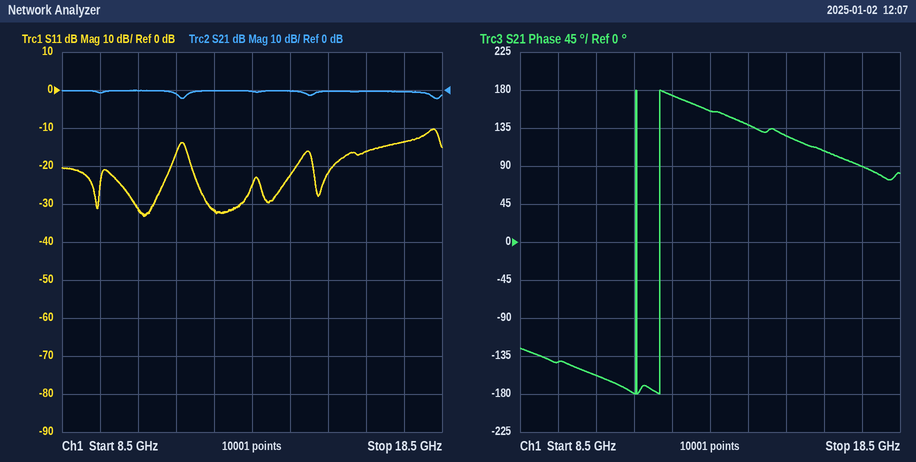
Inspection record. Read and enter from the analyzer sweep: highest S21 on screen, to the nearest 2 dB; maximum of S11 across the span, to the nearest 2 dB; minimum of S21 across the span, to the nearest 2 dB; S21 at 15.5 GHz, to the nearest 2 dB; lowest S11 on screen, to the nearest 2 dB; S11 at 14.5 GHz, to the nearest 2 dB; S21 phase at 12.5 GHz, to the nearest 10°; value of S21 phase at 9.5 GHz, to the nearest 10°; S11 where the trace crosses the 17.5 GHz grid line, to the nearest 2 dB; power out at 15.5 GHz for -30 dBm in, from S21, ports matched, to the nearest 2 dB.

0 dB
-10 dB
-2 dB
0 dB
-34 dB
-22 dB
170°
-140°
-14 dB
-30 dBm
